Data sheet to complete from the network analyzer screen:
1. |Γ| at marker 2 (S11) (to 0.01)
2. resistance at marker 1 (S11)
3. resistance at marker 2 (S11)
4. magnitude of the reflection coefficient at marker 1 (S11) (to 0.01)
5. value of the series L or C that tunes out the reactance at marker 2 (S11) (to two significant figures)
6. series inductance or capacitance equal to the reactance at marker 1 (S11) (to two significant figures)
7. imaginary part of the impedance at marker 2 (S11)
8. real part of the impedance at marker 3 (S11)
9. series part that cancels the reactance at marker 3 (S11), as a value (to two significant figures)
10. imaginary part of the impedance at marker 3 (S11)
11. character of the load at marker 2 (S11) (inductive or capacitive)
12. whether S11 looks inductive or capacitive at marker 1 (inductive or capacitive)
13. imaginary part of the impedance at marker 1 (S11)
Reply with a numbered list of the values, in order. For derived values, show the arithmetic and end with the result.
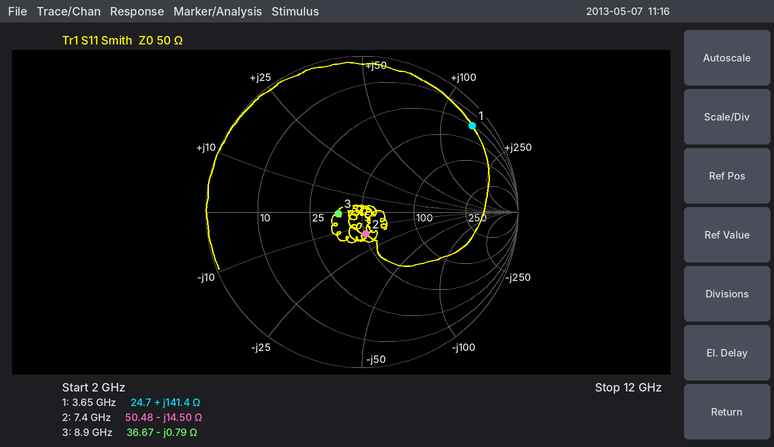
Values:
1. 0.14
2. 24.7 Ω
3. 50.48 Ω
4. 0.90
5. L = 14.5 Ω/(2π × 7.4 GHz) ≈ 312 pH, so 310 pH to two significant figures
6. L = 141.4 Ω/(2π × 3.65 GHz) ≈ 6.2 nH
7. -14.50 Ω
8. 36.67 Ω
9. L = 0.79 Ω/(2π × 8.9 GHz) ≈ 14 pH
10. -0.79 Ω
11. capacitive
12. inductive
13. +141.4 Ω
